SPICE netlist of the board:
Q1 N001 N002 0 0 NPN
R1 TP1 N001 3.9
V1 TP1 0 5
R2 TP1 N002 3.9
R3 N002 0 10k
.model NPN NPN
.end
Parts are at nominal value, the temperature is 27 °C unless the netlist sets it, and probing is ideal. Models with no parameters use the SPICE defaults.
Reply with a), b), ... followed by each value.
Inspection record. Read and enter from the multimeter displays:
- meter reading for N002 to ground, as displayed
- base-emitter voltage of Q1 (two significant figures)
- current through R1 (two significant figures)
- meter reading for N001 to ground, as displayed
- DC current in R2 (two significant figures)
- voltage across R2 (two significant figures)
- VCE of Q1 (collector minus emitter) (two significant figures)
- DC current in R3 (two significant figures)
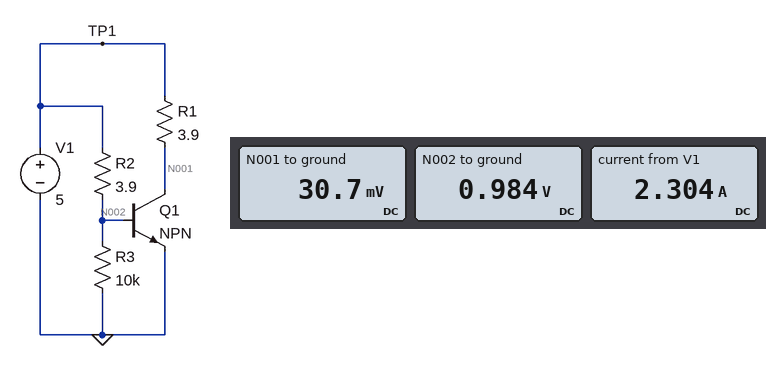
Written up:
a) 0.984 V
b) 980 mV
c) 1.3 A
d) 30.7 mV
e) 1.0 A
f) 4.0 V
g) 31 mV
h) 98 µA
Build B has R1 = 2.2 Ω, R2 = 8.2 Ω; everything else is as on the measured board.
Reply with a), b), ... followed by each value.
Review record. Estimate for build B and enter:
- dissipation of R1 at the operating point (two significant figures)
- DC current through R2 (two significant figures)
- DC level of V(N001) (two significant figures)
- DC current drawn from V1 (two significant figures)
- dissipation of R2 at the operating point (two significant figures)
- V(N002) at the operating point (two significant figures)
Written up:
a) 11 W
b) 490 mA
c) 50 mV
d) 2.7 A
e) 2.0 W
f) 980 mV
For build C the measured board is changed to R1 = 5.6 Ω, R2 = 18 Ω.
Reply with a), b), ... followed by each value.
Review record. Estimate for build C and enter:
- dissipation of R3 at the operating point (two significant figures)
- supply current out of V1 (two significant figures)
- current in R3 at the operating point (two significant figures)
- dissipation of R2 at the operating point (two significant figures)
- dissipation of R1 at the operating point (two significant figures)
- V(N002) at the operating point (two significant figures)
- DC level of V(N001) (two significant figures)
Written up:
a) 92 µW
b) 1.1 A
c) 96 µA
d) 910 mW
e) 4.4 W
f) 960 mV
g) 47 mV
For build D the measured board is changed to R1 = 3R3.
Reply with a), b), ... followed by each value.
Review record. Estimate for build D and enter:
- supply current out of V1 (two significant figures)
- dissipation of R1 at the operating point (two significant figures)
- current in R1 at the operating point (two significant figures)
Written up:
a) 2.5 A
b) 7.5 W
c) 1.5 A
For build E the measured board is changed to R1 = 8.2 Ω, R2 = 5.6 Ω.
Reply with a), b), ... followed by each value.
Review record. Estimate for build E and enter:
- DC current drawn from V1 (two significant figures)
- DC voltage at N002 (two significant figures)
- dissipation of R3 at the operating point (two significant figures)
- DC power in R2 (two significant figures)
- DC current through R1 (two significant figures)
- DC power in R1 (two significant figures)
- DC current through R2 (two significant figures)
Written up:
a) 1.3 A
b) 970 mV
c) 94 µW
d) 2.9 W
e) 610 mA
f) 3.0 W
g) 720 mA
